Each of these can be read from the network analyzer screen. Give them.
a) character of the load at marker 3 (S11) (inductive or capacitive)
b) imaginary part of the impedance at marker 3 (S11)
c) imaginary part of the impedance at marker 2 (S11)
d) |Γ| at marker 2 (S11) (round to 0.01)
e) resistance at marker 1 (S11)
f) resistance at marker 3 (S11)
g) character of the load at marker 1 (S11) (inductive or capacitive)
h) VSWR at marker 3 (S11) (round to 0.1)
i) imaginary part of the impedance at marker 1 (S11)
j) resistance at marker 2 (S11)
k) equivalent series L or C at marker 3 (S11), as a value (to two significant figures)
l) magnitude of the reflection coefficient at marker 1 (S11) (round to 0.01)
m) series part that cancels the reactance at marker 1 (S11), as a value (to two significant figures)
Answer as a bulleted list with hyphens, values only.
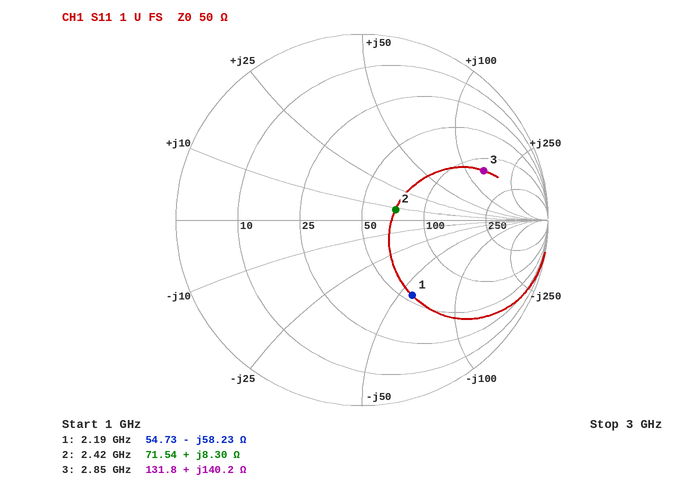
- inductive
- +140.2 Ω
- +8.30 Ω
- 0.19
- 54.73 Ω
- 131.8 Ω
- capacitive
- 5.8
- -58.23 Ω
- 71.54 Ω
- 7.8 nH
- 0.49
- 4.2 nH
